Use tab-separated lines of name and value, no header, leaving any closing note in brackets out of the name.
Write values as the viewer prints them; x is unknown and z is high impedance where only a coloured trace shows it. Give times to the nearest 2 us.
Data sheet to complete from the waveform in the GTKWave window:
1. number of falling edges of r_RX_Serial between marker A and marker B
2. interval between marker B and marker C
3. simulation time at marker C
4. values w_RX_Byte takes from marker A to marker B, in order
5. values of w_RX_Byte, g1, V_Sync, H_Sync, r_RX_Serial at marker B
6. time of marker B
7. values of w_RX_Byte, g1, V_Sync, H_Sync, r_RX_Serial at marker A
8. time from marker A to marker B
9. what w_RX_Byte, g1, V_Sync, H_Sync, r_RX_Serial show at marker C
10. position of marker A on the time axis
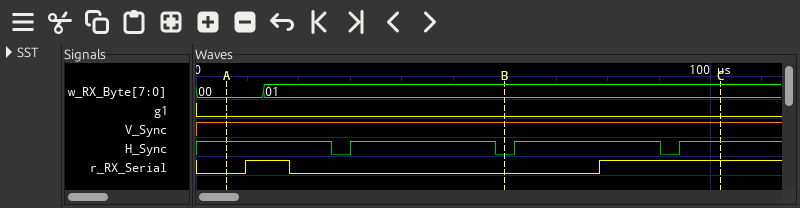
number of falling edges of r_RX_Serial between marker A and marker B	1
interval between marker B and marker C	42 us
simulation time at marker C	102 us
values w_RX_Byte takes from marker A to marker B, in order	00, 01
values of w_RX_Byte, g1, V_Sync, H_Sync, r_RX_Serial at marker B	w_RX_Byte=01, g1=0, V_Sync=1, H_Sync=0, r_RX_Serial=0
time of marker B	60 us
values of w_RX_Byte, g1, V_Sync, H_Sync, r_RX_Serial at marker A	w_RX_Byte=00, g1=0, V_Sync=1, H_Sync=1, r_RX_Serial=0
time from marker A to marker B	54 us
what w_RX_Byte, g1, V_Sync, H_Sync, r_RX_Serial show at marker C	w_RX_Byte=01, g1=0, V_Sync=1, H_Sync=1, r_RX_Serial=1
position of marker A on the time axis	6 us
